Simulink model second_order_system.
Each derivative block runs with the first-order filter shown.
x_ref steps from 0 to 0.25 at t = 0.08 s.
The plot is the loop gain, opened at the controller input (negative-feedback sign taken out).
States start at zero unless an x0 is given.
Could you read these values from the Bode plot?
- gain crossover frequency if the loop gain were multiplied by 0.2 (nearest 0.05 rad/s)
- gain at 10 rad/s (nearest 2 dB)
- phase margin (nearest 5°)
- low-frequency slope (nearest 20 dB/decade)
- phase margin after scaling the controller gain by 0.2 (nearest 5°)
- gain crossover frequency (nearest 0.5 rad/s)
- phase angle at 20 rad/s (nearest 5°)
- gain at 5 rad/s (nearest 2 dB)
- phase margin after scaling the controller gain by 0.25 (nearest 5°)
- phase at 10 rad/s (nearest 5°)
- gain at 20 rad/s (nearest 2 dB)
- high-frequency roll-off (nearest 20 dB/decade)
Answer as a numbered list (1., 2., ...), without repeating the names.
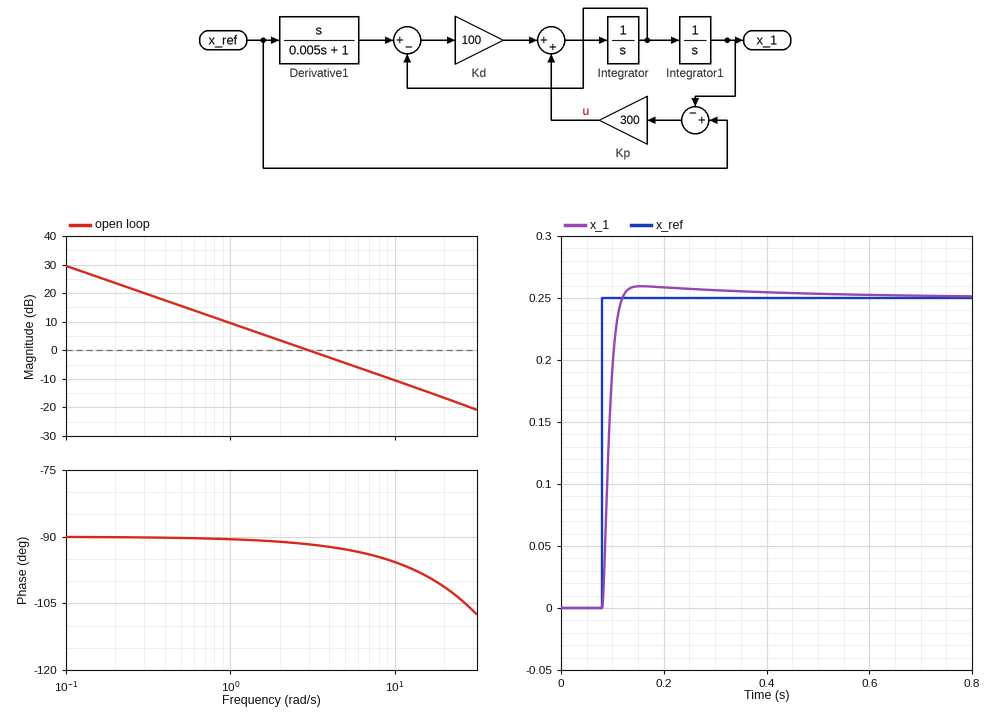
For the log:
1. 0.60 rad/s
2. -10 dB
3. 90°
4. -20 dB/decade
5. 90°
6. 3.0 rad/s
7. -100°
8. -4 dB
9. 90°
10. -95°
11. -16 dB
12. -20 dB/decade
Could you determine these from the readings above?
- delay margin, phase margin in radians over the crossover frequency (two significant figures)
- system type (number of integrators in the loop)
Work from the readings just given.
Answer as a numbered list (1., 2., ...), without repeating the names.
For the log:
1. 0.52 s
2. 1
